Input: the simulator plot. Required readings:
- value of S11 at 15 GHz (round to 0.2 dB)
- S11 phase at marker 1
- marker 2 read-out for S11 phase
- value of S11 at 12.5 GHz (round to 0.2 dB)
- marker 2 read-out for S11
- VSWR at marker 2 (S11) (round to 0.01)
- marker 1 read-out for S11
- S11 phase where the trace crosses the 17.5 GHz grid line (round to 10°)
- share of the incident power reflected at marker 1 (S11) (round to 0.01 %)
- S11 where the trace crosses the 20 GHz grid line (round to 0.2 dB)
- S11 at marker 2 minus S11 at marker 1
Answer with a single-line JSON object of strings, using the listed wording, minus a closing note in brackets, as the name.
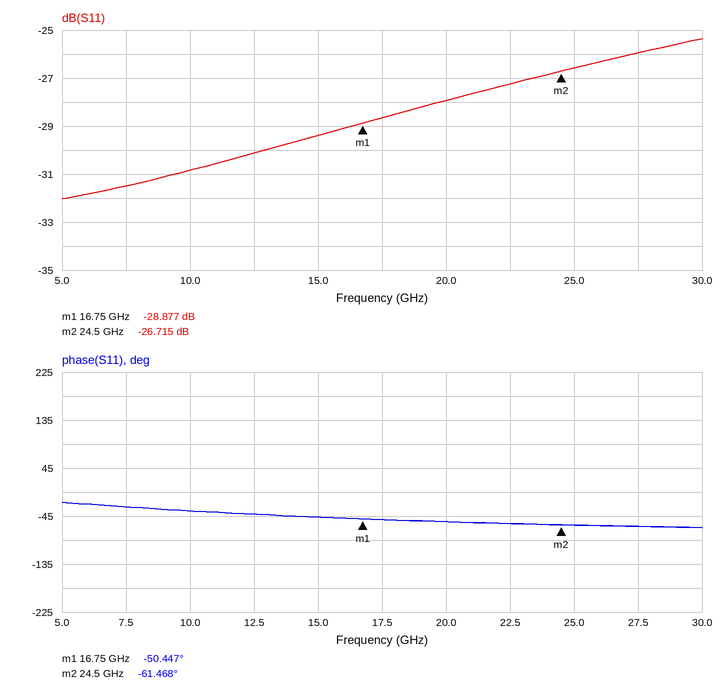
{"value of S11 at 15 GHz": "-29.4 dB", "S11 phase at marker 1": "-50.447°", "marker 2 read-out for S11 phase": "-61.468°", "value of S11 at 12.5 GHz": "-30.2 dB", "marker 2 read-out for S11": "-26.715 dB", "VSWR at marker 2 (S11)": "1.10", "marker 1 read-out for S11": "-28.877 dB", "S11 phase where the trace crosses the 17.5 GHz grid line": "-50°", "share of the incident power reflected at marker 1 (S11)": "0.13 %", "S11 where the trace crosses the 20 GHz grid line": "-28.0 dB", "S11 at marker 2 minus S11 at marker 1": "2.162 dB"}
